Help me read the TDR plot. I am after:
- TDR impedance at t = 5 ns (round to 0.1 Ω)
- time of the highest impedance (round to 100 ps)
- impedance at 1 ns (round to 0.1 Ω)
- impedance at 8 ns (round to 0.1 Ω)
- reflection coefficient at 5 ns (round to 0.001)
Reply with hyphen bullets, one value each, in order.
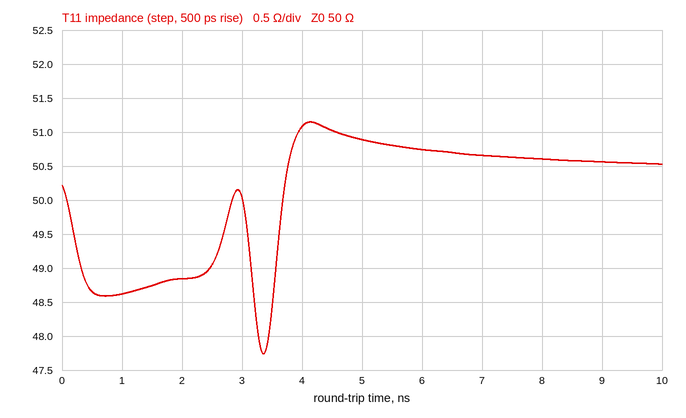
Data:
- 50.9 Ω
- 4.1 ns
- 48.6 Ω
- 50.6 Ω
- +0.009
